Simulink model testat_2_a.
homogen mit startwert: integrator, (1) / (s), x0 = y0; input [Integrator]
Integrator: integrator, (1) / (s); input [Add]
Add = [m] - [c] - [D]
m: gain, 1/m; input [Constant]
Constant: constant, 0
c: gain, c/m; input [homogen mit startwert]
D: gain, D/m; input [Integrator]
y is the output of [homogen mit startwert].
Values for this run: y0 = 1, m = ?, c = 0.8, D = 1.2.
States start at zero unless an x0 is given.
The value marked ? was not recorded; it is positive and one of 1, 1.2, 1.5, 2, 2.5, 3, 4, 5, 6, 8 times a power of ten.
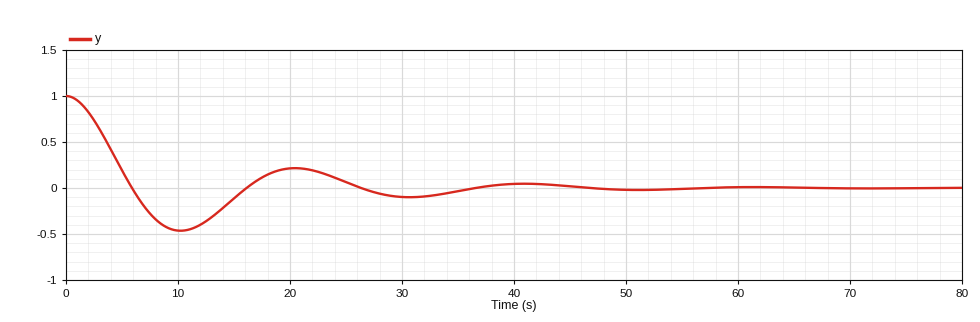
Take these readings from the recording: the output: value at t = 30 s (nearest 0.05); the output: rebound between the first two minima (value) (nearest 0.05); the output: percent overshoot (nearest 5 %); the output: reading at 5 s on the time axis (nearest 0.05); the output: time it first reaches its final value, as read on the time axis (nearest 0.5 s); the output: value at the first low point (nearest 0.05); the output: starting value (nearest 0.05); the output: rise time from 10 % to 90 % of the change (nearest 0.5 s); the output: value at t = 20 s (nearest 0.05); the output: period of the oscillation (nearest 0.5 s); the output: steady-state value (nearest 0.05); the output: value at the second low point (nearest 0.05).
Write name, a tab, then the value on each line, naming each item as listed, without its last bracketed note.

the output: value at t = 30 s	-0.10
the output: rebound between the first two minima (value)	0.20
the output: percent overshoot	45 %
the output: reading at 5 s on the time axis	0.20
the output: time it first reaches its final value, as read on the time axis	6.0 s
the output: value at the first low point	-0.45
the output: starting value	1.00
the output: rise time from 10 % to 90 % of the change	4.0 s
the output: value at t = 20 s	0.20
the output: period of the oscillation	20.5 s
the output: steady-state value	0.00
the output: value at the second low point	-0.10
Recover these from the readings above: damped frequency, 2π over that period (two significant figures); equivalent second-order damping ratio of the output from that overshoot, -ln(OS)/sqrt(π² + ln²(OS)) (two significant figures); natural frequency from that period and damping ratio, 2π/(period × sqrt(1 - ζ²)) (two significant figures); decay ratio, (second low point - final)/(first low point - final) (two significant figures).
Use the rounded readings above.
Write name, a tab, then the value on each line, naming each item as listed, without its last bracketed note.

damped frequency, 2π over that period	0.31 rad/s
equivalent second-order damping ratio of the output from that overshoot, -ln(OS)/sqrt(π² + ln²(OS))	0.25
natural frequency from that period and damping ratio, 2π/(period × sqrt(1 - ζ²))	0.32 rad/s
decay ratio, (second low point - final)/(first low point - final)	0.22
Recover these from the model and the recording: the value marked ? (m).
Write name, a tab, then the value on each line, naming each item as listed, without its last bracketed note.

the value marked ?	8
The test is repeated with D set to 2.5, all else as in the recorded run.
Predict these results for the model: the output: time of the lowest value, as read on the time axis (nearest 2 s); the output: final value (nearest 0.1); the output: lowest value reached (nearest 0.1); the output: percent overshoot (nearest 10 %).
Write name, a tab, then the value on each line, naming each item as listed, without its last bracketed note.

the output: time of the lowest value, as read on the time axis	12 s
the output: final value	0.0
the output: lowest value reached	-0.2
the output: percent overshoot	20 %
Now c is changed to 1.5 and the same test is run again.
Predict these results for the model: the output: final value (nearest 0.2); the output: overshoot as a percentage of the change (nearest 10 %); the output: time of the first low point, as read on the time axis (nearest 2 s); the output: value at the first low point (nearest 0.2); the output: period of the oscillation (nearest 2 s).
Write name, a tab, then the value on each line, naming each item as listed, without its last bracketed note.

the output: final value	0.0
the output: overshoot as a percentage of the change	60 %
the output: time of the first low point, as read on the time axis	8 s
the output: value at the first low point	-0.6
the output: period of the oscillation	14 s
